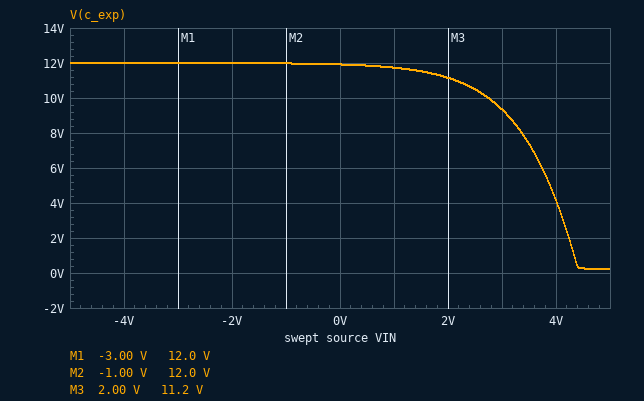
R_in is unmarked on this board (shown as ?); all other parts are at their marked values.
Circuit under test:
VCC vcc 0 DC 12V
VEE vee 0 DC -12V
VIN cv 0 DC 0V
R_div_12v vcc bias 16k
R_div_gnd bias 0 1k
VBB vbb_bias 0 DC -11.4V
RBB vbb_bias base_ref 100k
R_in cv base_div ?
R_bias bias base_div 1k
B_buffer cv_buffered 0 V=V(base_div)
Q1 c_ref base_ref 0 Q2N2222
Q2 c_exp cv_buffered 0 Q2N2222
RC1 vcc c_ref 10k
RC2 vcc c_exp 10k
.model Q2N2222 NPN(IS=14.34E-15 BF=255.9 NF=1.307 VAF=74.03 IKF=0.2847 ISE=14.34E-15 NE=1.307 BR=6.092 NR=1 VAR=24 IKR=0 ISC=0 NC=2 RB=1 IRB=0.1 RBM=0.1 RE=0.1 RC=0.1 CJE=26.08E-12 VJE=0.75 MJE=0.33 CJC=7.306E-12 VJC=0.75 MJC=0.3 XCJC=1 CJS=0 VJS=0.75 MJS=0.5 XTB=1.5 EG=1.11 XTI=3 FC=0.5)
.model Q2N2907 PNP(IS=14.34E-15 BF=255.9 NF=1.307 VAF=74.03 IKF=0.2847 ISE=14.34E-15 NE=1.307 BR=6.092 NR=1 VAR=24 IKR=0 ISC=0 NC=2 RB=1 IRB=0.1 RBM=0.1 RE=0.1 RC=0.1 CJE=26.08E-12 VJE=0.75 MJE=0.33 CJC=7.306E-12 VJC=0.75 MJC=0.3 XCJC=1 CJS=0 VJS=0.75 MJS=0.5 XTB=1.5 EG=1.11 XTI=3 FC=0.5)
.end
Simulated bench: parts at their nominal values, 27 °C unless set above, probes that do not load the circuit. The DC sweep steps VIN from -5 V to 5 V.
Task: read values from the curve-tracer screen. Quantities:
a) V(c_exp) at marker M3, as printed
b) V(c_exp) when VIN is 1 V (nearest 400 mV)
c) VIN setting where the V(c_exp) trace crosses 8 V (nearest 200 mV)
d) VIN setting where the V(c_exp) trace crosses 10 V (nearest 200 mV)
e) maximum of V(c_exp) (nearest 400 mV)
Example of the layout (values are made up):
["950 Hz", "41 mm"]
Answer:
["11.2 V", "11.6 V", "3.4 V", "2.8 V", "12.0 V"]
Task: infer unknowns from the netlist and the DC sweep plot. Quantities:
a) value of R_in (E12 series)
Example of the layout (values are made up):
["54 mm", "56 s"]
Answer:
["47 kΩ"]
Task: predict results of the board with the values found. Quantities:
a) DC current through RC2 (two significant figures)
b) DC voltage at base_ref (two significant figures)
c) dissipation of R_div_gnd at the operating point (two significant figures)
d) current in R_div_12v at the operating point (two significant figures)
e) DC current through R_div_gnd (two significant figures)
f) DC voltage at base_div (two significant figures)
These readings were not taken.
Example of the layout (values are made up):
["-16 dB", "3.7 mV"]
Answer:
["8.2 µA", "-11 V", "480 µW", "710 µA", "690 µA", "680 mV"]
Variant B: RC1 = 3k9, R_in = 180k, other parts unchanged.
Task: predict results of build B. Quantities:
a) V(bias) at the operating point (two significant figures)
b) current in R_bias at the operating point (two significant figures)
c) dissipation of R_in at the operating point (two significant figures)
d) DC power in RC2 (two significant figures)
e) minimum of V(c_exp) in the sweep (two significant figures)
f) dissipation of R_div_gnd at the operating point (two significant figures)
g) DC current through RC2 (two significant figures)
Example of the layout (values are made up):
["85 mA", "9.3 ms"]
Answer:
["700 mV", "3.9 µA", "2.7 µW", "2.3 µW", "11 V", "490 µW", "15 µA"]
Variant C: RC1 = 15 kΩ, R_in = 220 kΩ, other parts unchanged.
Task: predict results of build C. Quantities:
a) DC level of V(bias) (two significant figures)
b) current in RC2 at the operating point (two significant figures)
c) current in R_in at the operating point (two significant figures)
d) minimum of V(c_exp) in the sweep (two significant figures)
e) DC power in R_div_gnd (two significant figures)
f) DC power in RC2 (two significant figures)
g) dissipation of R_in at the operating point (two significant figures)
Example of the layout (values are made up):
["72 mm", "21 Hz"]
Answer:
["700 mV", "16 µA", "3.2 µA", "11 V", "490 µW", "2.5 µW", "2.2 µW"]
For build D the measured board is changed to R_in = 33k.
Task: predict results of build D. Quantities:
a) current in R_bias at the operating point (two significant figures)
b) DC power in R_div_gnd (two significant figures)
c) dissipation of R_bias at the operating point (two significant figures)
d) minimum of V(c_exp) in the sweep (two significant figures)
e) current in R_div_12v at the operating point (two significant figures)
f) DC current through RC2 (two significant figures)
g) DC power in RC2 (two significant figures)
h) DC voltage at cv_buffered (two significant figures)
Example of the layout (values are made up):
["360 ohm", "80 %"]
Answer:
["20 µA", "470 µW", "410 nW", "220 mV", "710 µA", "5.9 µA", "350 nW", "670 mV"]
